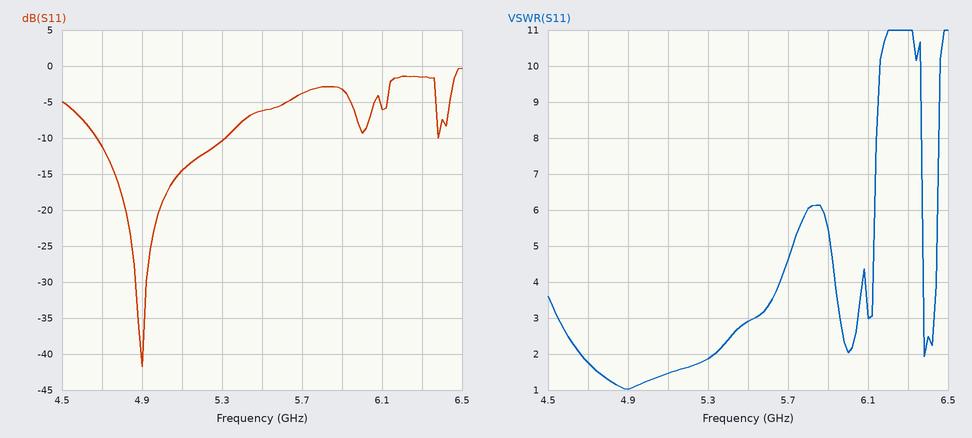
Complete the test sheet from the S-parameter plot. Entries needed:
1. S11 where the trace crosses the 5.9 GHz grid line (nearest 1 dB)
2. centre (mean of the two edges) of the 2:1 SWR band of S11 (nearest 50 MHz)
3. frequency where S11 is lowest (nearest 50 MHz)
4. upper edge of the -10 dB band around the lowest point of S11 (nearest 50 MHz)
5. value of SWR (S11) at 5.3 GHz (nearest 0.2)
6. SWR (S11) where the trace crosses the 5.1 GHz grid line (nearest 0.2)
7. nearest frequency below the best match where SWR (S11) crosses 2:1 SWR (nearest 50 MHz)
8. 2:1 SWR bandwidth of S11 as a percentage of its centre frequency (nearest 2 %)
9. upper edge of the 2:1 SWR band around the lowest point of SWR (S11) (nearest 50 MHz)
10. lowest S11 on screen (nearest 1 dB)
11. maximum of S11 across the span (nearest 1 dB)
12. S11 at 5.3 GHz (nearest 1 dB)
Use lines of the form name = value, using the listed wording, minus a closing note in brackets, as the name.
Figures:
S11 where the trace crosses the 5.9 GHz grid line = -3 dB
centre (mean of the two edges) of the 2:1 SWR band of S11 = 5.00 GHz
frequency where S11 is lowest = 4.90 GHz
upper edge of the -10 dB band around the lowest point of S11 = 5.30 GHz
value of SWR (S11) at 5.3 GHz = 1.8
SWR (S11) where the trace crosses the 5.1 GHz grid line = 1.4
nearest frequency below the best match where SWR (S11) crosses 2:1 SWR = 4.65 GHz
2:1 SWR bandwidth of S11 as a percentage of its centre frequency = 14 %
upper edge of the 2:1 SWR band around the lowest point of SWR (S11) = 5.35 GHz
lowest S11 on screen = -42 dB
maximum of S11 across the span = 0 dB
S11 at 5.3 GHz = -10 dB
